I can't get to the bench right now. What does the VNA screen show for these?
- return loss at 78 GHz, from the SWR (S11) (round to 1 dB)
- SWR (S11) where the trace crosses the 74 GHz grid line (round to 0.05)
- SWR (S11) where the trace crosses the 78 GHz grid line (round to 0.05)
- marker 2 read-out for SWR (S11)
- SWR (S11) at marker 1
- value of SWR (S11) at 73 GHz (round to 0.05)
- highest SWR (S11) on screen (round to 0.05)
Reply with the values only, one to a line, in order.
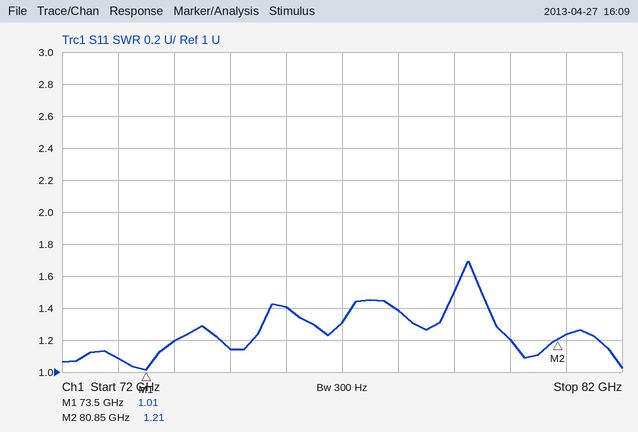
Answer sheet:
16 dB
1.20
1.40
1.21
1.01
1.10
1.70
